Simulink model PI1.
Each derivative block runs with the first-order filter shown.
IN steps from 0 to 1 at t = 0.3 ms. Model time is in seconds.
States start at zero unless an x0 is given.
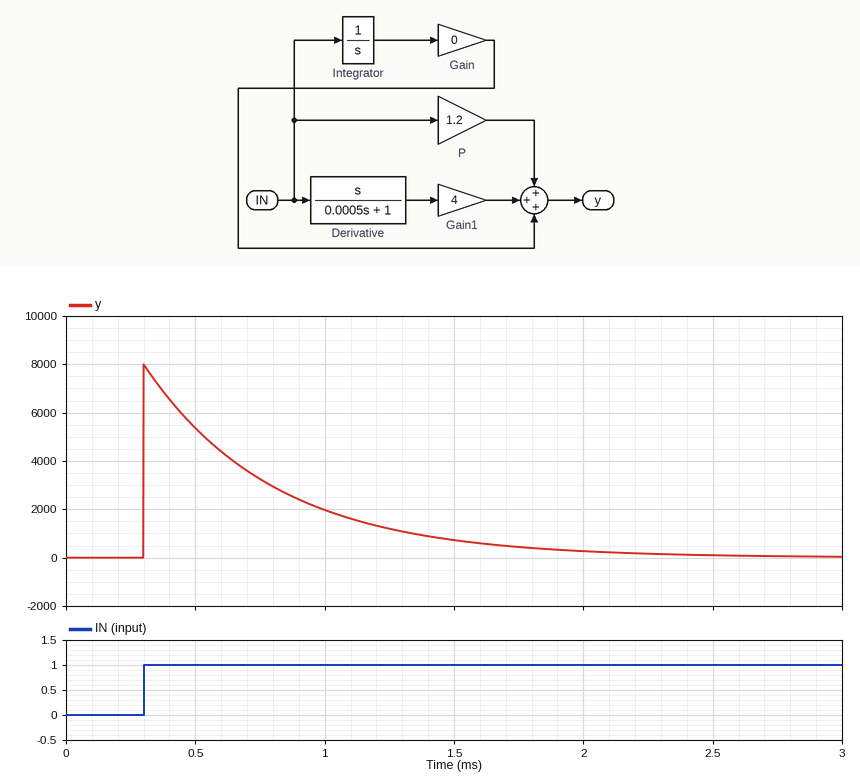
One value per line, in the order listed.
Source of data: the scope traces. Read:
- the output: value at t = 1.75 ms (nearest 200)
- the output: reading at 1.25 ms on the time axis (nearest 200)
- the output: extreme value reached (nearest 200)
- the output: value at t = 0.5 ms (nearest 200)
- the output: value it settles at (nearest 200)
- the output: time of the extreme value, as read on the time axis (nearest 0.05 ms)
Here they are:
400
1200
8000
5400
0
0.30 ms
